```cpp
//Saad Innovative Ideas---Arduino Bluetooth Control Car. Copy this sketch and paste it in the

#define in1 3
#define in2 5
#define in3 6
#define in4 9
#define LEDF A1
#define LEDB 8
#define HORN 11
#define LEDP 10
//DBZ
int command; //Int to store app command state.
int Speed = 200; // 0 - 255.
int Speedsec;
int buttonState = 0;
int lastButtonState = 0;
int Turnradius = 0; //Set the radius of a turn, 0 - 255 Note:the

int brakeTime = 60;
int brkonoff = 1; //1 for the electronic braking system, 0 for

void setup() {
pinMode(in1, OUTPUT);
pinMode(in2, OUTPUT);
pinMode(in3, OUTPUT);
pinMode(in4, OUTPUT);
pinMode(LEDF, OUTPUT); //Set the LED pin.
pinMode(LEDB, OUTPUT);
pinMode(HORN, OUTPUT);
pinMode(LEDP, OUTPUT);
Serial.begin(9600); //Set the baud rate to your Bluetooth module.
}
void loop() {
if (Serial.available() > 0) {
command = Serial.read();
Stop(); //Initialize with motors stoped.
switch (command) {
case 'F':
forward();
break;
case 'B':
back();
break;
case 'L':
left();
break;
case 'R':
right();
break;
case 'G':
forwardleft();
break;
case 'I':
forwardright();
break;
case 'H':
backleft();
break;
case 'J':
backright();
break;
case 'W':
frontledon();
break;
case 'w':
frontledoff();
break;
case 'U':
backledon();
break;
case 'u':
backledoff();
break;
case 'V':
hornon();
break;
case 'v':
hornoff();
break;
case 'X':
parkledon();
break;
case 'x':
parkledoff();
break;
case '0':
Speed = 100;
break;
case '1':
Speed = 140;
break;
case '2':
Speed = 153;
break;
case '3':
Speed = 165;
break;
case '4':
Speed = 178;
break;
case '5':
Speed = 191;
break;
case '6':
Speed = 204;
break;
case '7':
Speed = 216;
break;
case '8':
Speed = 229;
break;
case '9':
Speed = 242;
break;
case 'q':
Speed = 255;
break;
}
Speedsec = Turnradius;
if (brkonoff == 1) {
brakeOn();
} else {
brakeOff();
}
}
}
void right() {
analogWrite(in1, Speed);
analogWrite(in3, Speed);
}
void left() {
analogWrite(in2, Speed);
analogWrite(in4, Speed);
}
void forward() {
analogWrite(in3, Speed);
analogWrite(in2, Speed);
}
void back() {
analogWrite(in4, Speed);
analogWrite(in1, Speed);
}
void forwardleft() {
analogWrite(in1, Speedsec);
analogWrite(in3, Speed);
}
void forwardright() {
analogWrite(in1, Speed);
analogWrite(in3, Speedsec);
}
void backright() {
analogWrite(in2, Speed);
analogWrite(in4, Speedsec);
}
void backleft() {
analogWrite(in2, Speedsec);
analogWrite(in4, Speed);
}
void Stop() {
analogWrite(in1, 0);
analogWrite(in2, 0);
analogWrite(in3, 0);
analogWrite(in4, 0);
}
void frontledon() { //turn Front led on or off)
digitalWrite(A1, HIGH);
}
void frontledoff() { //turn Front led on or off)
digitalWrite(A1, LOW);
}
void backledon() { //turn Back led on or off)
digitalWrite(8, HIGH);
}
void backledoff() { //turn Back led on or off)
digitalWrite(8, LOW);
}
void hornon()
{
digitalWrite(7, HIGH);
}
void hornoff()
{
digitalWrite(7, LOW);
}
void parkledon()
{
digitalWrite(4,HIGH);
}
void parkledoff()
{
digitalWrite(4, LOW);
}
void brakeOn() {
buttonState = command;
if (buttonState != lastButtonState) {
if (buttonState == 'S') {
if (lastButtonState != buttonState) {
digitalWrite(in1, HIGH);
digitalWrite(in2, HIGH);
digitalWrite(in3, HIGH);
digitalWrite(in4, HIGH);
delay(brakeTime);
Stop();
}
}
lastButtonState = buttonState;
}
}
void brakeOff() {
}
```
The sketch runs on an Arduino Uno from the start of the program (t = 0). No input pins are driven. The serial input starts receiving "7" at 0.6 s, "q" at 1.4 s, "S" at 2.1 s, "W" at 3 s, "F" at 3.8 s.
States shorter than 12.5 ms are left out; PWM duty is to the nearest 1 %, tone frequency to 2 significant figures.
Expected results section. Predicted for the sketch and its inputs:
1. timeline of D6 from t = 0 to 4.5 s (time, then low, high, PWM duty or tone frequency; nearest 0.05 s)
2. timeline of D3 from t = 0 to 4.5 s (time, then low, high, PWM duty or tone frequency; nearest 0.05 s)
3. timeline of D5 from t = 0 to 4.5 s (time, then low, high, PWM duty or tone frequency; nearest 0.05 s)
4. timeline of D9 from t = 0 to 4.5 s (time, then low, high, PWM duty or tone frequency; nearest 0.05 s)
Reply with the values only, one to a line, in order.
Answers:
0 s low; 2.1 s high; 2.15 s low; 3.8 s high
0 s low; 2.1 s high; 2.15 s low
0 s low; 2.1 s high; 2.15 s low; 3.8 s high
0 s low; 2.1 s high; 2.15 s low
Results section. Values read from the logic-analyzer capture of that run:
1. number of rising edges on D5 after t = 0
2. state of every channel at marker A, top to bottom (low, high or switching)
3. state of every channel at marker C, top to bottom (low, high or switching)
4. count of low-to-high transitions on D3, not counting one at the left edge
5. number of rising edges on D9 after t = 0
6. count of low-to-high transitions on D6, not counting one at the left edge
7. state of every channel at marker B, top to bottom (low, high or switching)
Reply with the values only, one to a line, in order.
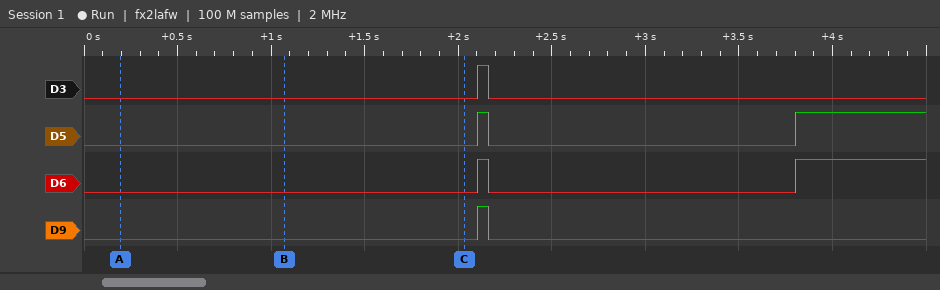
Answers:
2
D3 low, D5 low, D6 low, D9 low
D3 low, D5 low, D6 low, D9 low
1
1
2
D3 low, D5 low, D6 low, D9 low
